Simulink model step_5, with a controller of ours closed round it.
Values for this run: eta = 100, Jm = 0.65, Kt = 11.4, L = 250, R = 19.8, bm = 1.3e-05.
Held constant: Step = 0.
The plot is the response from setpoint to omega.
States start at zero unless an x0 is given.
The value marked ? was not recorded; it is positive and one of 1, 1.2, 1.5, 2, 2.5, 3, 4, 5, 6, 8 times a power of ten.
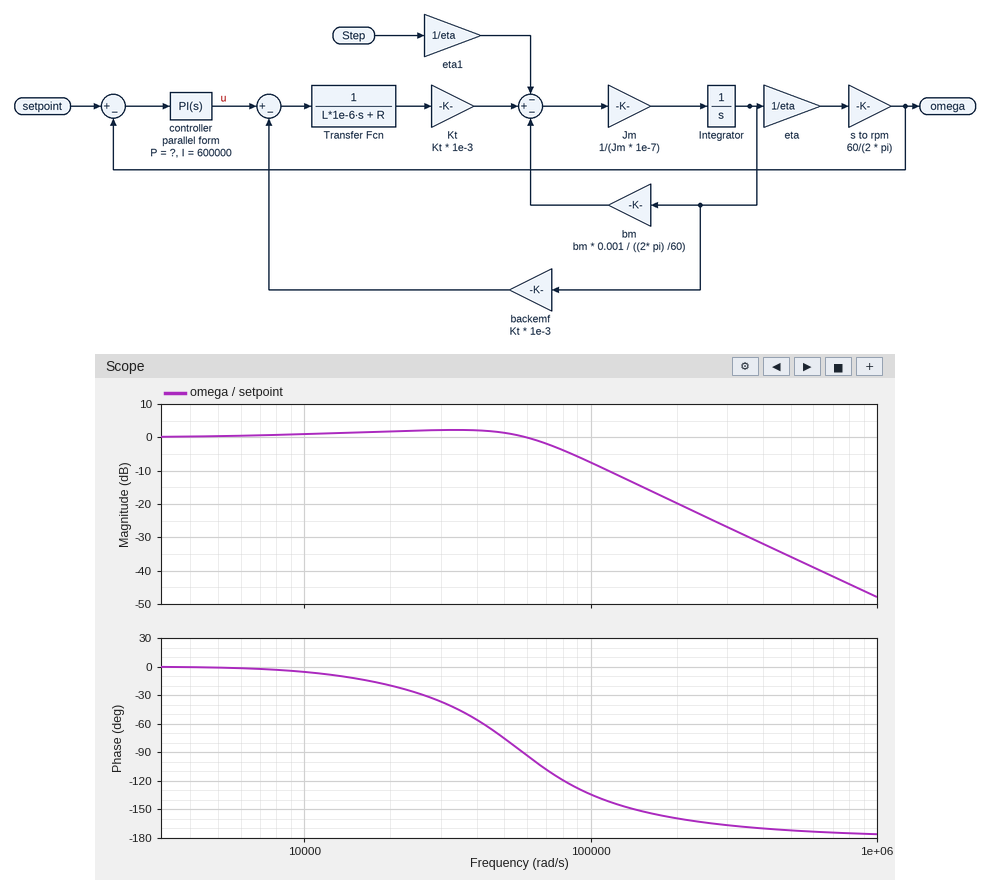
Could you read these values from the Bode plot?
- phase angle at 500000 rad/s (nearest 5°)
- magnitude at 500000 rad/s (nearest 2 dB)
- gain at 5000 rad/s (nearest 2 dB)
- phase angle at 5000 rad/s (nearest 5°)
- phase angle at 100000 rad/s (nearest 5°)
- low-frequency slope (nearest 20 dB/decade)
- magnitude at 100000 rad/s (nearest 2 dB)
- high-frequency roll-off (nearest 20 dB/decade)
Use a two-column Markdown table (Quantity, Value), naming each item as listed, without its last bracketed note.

| Quantity | Value |
|---|---|
| phase angle at 500000 rad/s | -170° |
| magnitude at 500000 rad/s | -36 dB |
| gain at 5000 rad/s | 0 dB |
| phase angle at 5000 rad/s | 0° |
| phase angle at 100000 rad/s | -135° |
| low-frequency slope | 0 dB/decade |
| magnitude at 100000 rad/s | -8 dB |
| high-frequency roll-off | -40 dB/decade |
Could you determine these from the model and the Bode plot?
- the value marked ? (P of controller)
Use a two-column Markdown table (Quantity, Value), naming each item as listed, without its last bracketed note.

| Quantity | Value |
|---|---|
| the value marked ? | 60 |
